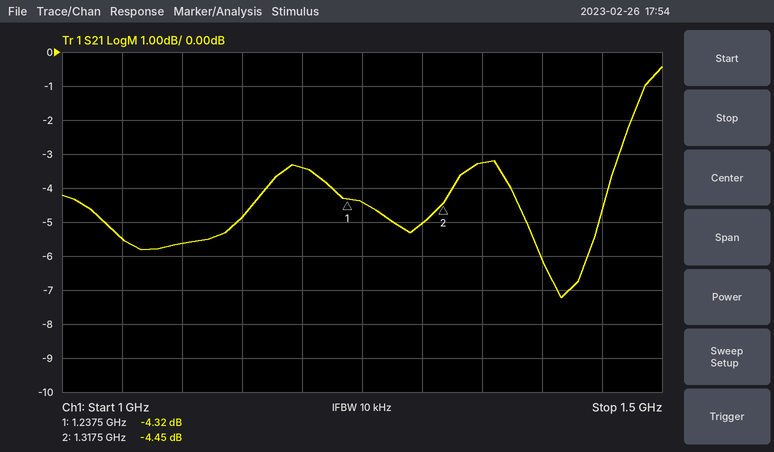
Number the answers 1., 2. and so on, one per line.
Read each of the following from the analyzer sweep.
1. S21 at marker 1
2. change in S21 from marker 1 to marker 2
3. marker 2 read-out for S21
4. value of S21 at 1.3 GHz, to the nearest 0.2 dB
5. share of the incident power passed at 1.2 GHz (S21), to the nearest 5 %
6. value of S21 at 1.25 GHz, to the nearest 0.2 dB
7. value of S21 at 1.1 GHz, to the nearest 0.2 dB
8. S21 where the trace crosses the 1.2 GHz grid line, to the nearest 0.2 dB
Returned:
1. -4.32 dB
2. -0.13 dB
3. -4.45 dB
4. -5.0 dB
5. 45 %
6. -4.4 dB
7. -5.6 dB
8. -3.4 dB
